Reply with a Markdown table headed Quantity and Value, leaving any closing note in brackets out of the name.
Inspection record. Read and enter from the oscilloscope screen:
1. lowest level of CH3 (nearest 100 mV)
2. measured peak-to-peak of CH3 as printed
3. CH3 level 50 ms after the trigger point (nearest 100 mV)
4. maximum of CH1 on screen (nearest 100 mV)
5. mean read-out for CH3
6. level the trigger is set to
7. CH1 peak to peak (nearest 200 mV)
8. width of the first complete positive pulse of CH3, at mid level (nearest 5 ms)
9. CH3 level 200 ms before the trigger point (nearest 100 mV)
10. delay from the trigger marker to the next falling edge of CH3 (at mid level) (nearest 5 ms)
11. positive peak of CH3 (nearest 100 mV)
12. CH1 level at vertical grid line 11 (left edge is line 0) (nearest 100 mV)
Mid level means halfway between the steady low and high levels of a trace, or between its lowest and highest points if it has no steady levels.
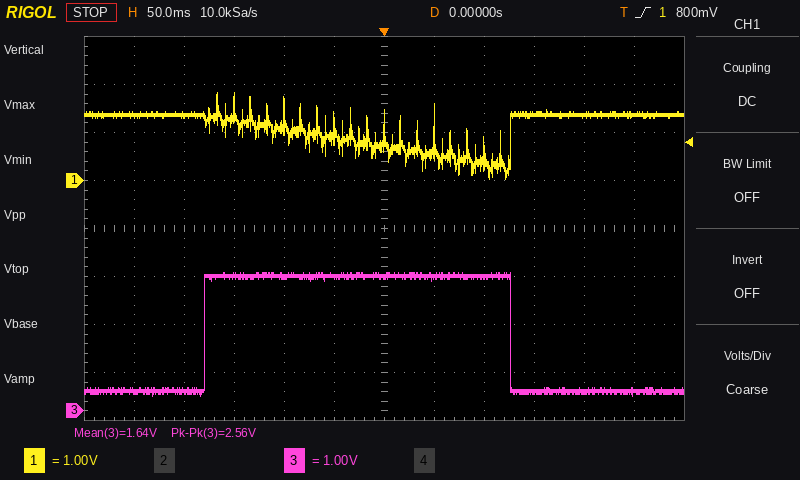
| Quantity | Value |
|---|---|
| lowest level of CH3 | 300 mV |
| measured peak-to-peak of CH3 as printed | 2.56 V |
| CH3 level 50 ms after the trigger point | 2.8 V |
| maximum of CH1 on screen | 1.8 V |
| mean read-out for CH3 | 1.64 V |
| level the trigger is set to | 800 mV |
| CH1 peak to peak | 1.8 V |
| width of the first complete positive pulse of CH3, at mid level | 305 ms |
| CH3 level 200 ms before the trigger point | 400 mV |
| delay from the trigger marker to the next falling edge of CH3 (at mid level) | 125 ms |
| positive peak of CH3 | 2.9 V |
| CH1 level at vertical grid line 11 (left edge is line 0) | 1.4 V |
